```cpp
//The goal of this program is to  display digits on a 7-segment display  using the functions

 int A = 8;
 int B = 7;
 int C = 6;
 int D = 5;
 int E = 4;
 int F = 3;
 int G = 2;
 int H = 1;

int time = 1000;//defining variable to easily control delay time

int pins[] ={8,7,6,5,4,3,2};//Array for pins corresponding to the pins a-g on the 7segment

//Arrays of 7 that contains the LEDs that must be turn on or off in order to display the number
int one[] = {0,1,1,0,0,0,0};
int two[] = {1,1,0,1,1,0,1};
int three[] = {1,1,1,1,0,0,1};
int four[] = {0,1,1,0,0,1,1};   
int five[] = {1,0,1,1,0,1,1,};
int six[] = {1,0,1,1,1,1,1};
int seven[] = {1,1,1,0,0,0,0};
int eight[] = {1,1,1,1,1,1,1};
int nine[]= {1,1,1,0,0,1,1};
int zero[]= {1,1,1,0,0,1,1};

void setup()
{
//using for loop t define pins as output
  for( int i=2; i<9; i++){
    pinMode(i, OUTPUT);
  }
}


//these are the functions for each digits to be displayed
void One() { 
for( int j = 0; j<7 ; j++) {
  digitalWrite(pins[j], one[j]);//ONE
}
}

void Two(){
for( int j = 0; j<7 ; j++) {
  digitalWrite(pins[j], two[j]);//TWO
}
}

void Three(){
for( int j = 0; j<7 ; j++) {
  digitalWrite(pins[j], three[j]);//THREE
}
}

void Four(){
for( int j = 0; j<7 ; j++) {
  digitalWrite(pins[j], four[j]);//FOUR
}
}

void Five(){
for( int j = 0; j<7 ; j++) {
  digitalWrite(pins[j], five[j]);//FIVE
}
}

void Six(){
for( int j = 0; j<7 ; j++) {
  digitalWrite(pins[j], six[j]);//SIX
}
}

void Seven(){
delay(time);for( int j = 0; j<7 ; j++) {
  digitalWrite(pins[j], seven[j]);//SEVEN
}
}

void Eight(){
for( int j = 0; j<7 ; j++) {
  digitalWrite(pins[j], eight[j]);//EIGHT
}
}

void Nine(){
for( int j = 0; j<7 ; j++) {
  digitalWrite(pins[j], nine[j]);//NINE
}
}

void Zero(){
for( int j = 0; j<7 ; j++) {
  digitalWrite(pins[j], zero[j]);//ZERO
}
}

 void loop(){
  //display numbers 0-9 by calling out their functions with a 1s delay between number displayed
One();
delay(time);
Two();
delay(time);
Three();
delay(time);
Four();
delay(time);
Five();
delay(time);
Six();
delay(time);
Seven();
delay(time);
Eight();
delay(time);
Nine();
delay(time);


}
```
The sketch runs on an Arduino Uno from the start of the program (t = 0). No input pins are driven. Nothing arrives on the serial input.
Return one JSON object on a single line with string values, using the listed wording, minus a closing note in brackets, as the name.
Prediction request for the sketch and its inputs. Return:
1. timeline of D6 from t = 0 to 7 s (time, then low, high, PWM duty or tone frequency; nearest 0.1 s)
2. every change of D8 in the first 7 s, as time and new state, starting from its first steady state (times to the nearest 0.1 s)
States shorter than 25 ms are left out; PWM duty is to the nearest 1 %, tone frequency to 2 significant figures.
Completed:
{"timeline of D6 from t = 0 to 7 s": "0 s high; 1 s low; 2 s high", "every change of D8 in the first 7 s, as time and new state, starting from its first steady state": "0 s low; 1 s high; 3 s low; 4 s high"}
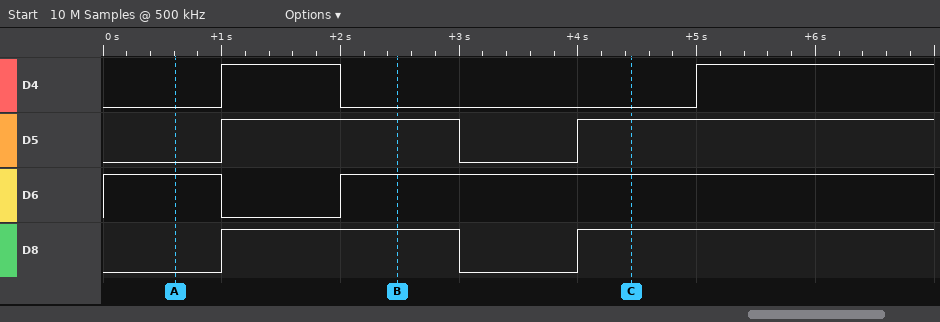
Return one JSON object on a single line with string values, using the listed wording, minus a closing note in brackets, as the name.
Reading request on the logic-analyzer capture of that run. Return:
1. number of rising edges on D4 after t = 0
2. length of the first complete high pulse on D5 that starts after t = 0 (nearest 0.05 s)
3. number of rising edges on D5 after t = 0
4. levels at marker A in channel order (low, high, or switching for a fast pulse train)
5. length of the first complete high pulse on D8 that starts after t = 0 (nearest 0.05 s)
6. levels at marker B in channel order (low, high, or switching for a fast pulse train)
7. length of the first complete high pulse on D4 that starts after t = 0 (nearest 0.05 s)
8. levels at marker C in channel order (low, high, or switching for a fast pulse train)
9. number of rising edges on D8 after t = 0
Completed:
{"number of rising edges on D4 after t = 0": "2", "length of the first complete high pulse on D5 that starts after t = 0": "2.00 s", "number of rising edges on D5 after t = 0": "2", "levels at marker A in channel order": "D4 low, D5 low, D6 high, D8 low", "length of the first complete high pulse on D8 that starts after t = 0": "2.00 s", "levels at marker B in channel order": "D4 low, D5 high, D6 high, D8 high", "length of the first complete high pulse on D4 that starts after t = 0": "1.00 s", "levels at marker C in channel order": "D4 low, D5 high, D6 high, D8 high", "number of rising edges on D8 after t = 0": "2"}
